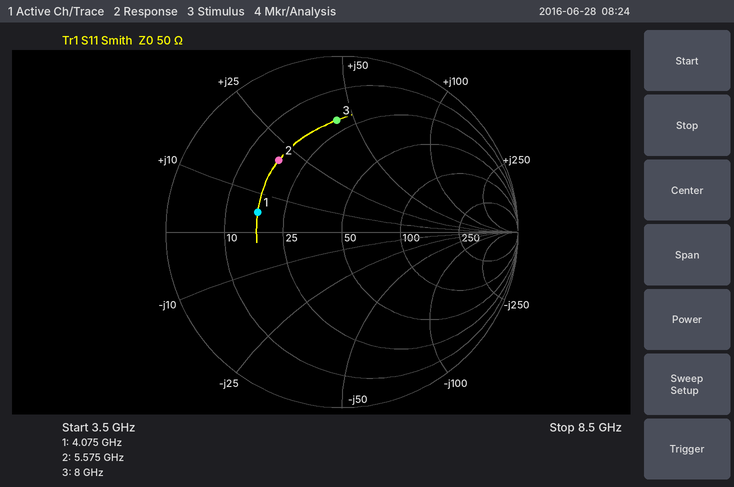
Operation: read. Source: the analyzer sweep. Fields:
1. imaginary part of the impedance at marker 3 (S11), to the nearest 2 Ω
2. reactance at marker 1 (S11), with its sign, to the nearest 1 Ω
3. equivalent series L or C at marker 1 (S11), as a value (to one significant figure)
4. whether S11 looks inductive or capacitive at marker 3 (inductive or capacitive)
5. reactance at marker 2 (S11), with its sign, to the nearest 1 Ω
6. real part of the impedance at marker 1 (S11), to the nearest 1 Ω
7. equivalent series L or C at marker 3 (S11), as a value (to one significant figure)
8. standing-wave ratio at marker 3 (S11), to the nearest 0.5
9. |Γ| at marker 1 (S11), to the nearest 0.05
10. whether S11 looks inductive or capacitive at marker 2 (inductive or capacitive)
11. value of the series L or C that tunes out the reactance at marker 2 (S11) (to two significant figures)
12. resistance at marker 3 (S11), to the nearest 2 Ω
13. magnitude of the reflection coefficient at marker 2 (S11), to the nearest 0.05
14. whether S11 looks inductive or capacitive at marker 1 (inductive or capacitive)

+44 Ω
+5 Ω
200 pH
inductive
+20 Ω
17 Ω
900 pH
4.5
0.50
inductive
1.4 pF
20 Ω
0.55
inductive
